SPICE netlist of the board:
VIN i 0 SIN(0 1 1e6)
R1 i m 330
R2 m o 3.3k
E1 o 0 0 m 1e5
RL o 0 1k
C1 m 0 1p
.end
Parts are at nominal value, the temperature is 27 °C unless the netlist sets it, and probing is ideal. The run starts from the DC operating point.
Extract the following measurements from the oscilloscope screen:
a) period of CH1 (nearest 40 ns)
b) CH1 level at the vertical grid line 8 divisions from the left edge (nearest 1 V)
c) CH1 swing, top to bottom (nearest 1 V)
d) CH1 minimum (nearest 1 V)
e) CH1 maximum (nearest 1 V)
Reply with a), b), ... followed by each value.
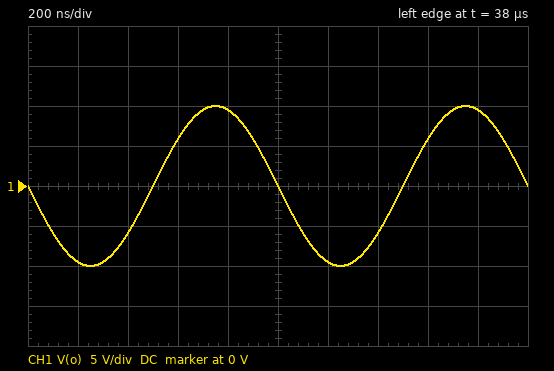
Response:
a) 1.00 µs
b) 6 V
c) 20 V
d) -10 V
e) 10 V
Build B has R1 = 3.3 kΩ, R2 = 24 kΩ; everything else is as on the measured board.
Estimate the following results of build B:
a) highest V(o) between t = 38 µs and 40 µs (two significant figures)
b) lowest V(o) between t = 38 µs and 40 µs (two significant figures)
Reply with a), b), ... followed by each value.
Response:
a) 7.3 V
b) -7.3 V
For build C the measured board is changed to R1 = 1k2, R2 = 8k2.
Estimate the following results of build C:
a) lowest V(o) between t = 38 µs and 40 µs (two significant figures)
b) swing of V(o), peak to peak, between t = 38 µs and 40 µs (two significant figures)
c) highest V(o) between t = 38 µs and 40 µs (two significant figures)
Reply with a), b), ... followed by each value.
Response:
a) -6.8 V
b) 14 V
c) 6.8 V
